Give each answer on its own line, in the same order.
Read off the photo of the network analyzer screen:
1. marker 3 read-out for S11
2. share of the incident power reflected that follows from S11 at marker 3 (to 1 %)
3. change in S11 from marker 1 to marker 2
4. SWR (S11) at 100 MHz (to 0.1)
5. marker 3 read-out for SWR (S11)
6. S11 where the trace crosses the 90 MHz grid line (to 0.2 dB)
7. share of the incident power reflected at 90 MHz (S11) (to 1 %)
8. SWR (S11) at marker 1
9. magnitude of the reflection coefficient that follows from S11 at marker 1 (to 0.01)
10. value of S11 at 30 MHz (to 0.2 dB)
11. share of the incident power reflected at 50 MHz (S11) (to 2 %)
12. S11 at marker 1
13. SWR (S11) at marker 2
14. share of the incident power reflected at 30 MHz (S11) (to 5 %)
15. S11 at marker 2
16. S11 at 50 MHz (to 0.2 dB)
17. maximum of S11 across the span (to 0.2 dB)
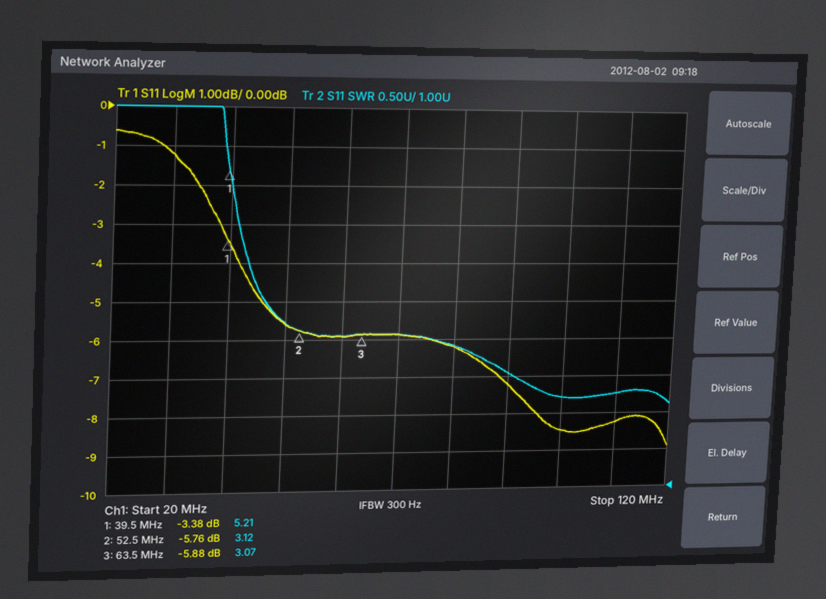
-5.88 dB
26 %
-2.38 dB
2.2
3.07
-7.2 dB
19 %
5.21
0.68
-1.2 dB
28 %
-3.38 dB
3.12
75 %
-5.76 dB
-5.6 dB
-0.6 dB
